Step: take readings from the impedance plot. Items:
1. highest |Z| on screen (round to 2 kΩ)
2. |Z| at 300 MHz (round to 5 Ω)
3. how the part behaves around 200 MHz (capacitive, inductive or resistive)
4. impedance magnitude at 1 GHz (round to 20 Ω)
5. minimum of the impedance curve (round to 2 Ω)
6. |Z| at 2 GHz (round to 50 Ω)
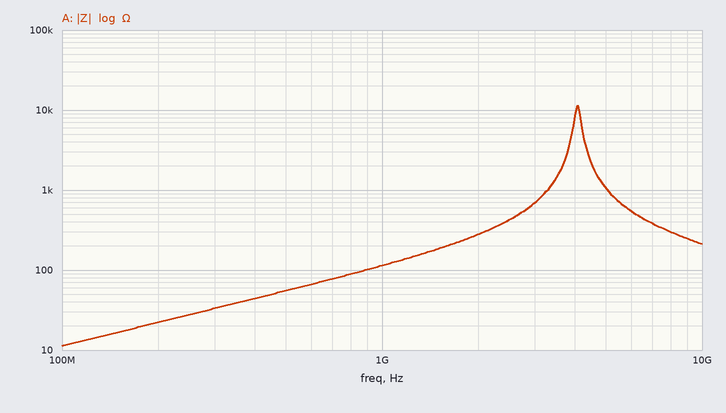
12 kΩ
35 Ω
inductive
120 Ω
12 Ω
300 Ω
